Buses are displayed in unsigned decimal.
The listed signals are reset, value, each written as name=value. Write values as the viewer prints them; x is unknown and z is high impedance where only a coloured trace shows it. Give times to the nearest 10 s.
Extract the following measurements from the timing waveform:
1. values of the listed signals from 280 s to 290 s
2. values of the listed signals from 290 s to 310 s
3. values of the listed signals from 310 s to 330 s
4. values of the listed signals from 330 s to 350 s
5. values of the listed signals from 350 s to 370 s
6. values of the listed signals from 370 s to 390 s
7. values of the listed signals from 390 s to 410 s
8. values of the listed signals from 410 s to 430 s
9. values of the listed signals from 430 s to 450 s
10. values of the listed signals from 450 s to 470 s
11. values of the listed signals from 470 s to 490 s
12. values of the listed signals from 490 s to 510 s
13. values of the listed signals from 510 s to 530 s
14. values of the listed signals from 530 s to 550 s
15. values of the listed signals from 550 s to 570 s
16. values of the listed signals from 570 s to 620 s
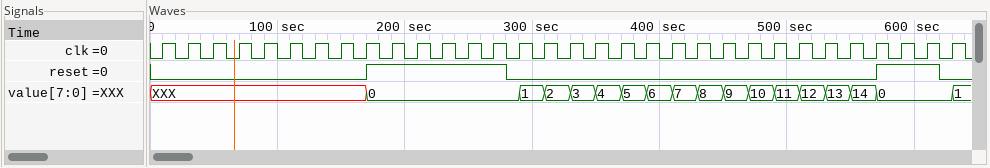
reset=0, value=0
reset=0, value=1
reset=0, value=2
reset=0, value=3
reset=0, value=4
reset=0, value=5
reset=0, value=6
reset=0, value=7
reset=0, value=8
reset=0, value=9
reset=0, value=10
reset=0, value=11
reset=0, value=12
reset=0, value=13
reset=0, value=14
reset=1, value=0
